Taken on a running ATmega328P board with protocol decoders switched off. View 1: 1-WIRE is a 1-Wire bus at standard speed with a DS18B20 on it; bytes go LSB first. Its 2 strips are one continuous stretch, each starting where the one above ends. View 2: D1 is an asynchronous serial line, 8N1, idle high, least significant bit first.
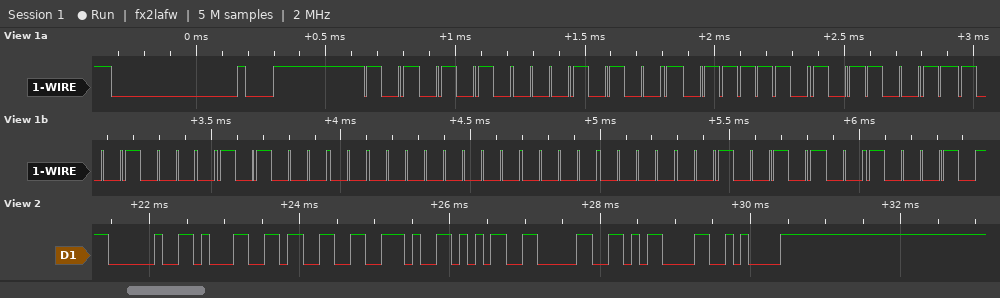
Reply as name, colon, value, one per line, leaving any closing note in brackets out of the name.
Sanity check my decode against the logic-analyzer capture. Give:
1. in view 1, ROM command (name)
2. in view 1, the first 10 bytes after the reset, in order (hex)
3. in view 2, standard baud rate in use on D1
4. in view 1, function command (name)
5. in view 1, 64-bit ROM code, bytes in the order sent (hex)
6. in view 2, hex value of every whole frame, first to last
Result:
in view 1, ROM command: Match ROM
in view 1, the first 10 bytes after the reset, in order: 55 28 7D CD 09 05 00 00 A4 44
in view 2, standard baud rate in use on D1: 9600 baud
in view 1, function command: Convert T
in view 1, 64-bit ROM code, bytes in the order sent: 28 7D CD 09 05 00 00 A4
in view 2, hex value of every whole frame, first to last: 20 31 33 2E 35 30 0D 0A
